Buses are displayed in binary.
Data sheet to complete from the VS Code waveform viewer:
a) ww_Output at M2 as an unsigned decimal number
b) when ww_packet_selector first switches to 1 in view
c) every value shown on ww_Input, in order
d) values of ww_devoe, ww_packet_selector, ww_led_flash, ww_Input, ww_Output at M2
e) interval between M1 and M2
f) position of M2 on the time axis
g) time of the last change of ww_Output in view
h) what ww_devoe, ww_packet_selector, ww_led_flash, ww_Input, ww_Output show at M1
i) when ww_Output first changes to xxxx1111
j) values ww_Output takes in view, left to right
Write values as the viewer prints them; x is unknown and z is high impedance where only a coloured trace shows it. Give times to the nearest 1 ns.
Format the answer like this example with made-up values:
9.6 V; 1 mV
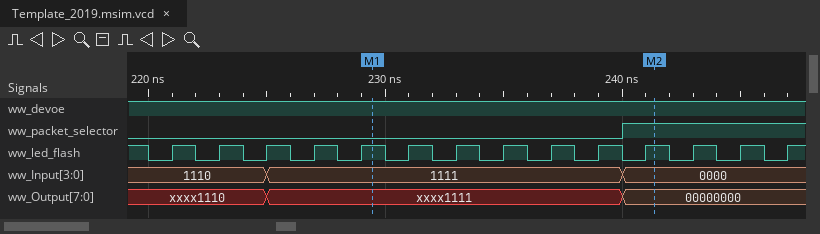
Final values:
0; 240 ns; 1110, 1111, 0000; ww_devoe=1, ww_packet_selector=1, ww_led_flash=1, ww_Input=0000, ww_Output=00000000; 12 ns; 241 ns; 240 ns; ww_devoe=1, ww_packet_selector=0, ww_led_flash=1, ww_Input=1111, ww_Output=xxxx1111; 225 ns; xxxx1110, xxxx1111, 00000000
